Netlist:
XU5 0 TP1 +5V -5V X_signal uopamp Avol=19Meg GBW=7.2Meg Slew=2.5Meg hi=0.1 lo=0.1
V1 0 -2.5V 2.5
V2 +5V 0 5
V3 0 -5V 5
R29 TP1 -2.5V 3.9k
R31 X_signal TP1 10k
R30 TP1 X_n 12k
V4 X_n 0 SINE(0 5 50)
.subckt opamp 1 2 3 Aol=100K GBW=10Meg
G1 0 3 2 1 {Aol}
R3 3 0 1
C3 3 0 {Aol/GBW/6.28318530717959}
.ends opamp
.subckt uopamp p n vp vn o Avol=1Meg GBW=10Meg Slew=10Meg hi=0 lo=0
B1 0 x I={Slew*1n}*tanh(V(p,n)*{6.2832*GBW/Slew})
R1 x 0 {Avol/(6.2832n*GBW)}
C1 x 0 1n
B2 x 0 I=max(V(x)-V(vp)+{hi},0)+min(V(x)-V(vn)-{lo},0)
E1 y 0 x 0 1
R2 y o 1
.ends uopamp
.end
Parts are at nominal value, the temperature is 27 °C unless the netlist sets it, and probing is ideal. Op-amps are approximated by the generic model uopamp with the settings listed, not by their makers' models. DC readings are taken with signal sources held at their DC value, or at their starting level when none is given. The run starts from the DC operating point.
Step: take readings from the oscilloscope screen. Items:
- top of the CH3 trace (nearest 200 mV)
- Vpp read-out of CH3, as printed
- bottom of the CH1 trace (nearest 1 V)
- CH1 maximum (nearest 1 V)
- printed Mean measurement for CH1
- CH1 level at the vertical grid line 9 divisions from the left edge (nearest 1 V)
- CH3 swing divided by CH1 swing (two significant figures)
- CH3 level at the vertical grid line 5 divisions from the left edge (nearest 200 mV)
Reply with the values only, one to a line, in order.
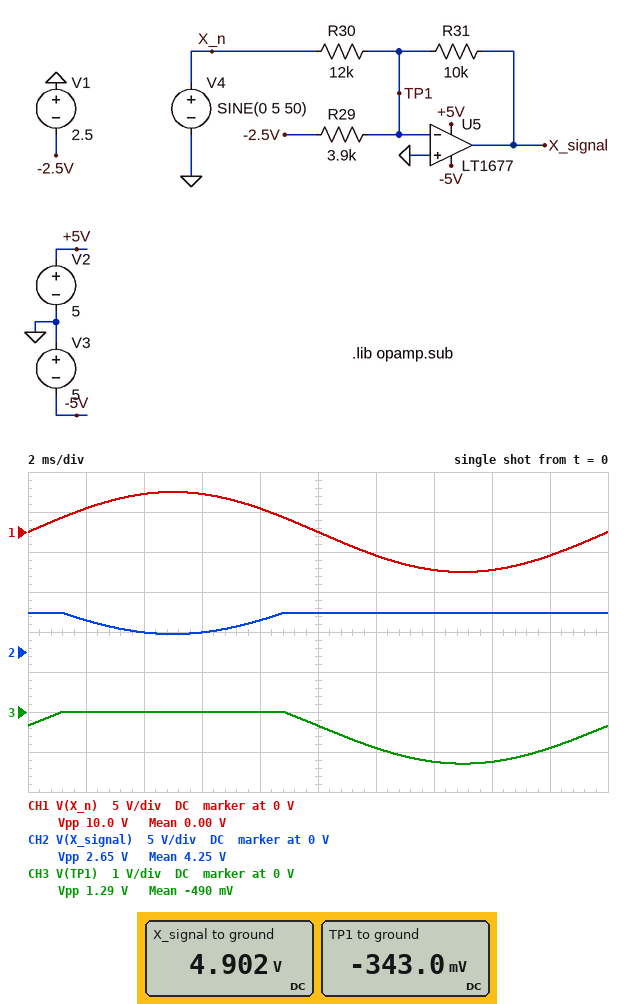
0 V
1.29 V
-5 V
5 V
0.00 V
-3 V
0.13
-400 mV
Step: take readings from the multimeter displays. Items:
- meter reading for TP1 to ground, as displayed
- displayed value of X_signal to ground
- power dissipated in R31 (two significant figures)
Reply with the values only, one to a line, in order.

-343.0 mV
4.902 V
2.8 mW
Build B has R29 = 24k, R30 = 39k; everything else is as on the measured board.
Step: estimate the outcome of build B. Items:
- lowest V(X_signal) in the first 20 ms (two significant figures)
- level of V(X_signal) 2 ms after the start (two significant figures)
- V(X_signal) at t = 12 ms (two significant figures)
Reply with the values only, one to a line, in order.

-240 mV
290 mV
1.8 V
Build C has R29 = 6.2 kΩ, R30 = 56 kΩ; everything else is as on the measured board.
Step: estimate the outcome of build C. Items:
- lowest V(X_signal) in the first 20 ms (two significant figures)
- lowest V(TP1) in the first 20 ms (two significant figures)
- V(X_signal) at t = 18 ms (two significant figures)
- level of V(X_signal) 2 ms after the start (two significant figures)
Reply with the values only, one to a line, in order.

3.1 V
-9.0 mV
4.6 V
3.5 V
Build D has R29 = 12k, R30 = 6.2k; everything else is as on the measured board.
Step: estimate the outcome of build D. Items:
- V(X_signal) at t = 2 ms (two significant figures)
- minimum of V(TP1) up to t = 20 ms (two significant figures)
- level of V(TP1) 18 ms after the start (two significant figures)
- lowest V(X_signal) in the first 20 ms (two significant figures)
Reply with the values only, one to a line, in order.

-2.7 V
-1.5 V
-560 mV
-4.9 V
